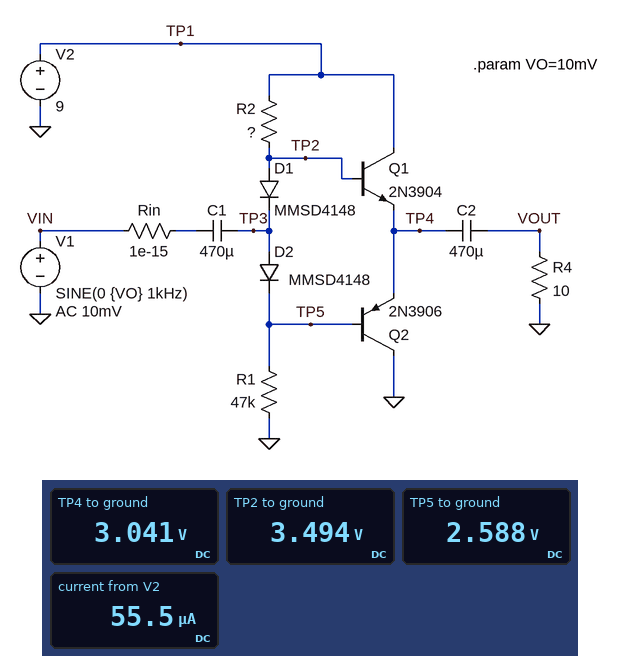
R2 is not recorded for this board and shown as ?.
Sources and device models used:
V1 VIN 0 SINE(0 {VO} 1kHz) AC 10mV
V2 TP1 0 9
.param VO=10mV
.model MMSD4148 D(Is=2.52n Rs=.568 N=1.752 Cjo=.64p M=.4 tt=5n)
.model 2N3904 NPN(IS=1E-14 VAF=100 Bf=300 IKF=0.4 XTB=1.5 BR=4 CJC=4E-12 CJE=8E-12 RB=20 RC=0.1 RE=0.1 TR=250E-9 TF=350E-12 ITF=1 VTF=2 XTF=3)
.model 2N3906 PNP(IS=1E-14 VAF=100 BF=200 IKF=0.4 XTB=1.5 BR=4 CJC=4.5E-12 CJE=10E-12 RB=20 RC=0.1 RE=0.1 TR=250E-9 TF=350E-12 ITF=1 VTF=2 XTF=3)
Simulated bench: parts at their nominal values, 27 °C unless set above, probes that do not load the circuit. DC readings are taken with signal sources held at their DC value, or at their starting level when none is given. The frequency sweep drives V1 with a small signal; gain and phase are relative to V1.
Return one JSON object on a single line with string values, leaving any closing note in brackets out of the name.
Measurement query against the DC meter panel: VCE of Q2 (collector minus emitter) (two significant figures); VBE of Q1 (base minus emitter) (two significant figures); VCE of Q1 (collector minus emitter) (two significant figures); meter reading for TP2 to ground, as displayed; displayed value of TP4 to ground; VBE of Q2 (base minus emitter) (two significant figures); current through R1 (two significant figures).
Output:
{"VCE of Q2 (collector minus emitter)": "-3.0 V", "VBE of Q1 (base minus emitter)": "450 mV", "VCE of Q1 (collector minus emitter)": "6.0 V", "meter reading for TP2 to ground, as displayed": "3.494 V", "displayed value of TP4 to ground": "3.041 V", "VBE of Q2 (base minus emitter)": "-450 mV", "current through R1": "55 µA"}
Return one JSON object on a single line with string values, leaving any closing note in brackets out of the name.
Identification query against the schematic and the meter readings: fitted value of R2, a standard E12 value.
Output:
{"fitted value of R2, a standard E12 value": "100 kΩ"}
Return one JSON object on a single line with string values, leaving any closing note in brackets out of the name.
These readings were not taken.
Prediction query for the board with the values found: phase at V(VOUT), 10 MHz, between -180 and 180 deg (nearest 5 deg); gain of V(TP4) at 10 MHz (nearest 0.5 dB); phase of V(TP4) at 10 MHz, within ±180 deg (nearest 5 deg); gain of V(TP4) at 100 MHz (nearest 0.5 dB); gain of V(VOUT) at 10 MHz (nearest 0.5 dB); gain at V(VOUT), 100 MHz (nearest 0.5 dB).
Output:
{"phase at V(VOUT), 10 MHz, between -180 and 180 deg": "60 deg", "gain of V(TP4) at 10 MHz": "-39.5 dB", "phase of V(TP4) at 10 MHz, within ±180 deg": "60 deg", "gain of V(TP4) at 100 MHz": "-26.0 dB", "gain of V(VOUT) at 10 MHz": "-39.5 dB", "gain at V(VOUT), 100 MHz": "-26.0 dB"}
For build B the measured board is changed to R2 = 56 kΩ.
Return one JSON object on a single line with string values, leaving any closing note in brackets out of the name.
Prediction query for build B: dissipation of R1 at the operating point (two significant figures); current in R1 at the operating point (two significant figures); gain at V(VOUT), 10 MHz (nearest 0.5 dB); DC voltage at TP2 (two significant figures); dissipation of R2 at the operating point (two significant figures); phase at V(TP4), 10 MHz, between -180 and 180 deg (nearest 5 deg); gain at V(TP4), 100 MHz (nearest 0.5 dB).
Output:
{"dissipation of R1 at the operating point": "290 µW", "current in R1 at the operating point": "78 µA", "gain at V(VOUT), 10 MHz": "-38.5 dB", "DC voltage at TP2": "4.6 V", "dissipation of R2 at the operating point": "340 µW", "phase at V(TP4), 10 MHz, between -180 and 180 deg": "65 deg", "gain at V(TP4), 100 MHz": "-24.5 dB"}
